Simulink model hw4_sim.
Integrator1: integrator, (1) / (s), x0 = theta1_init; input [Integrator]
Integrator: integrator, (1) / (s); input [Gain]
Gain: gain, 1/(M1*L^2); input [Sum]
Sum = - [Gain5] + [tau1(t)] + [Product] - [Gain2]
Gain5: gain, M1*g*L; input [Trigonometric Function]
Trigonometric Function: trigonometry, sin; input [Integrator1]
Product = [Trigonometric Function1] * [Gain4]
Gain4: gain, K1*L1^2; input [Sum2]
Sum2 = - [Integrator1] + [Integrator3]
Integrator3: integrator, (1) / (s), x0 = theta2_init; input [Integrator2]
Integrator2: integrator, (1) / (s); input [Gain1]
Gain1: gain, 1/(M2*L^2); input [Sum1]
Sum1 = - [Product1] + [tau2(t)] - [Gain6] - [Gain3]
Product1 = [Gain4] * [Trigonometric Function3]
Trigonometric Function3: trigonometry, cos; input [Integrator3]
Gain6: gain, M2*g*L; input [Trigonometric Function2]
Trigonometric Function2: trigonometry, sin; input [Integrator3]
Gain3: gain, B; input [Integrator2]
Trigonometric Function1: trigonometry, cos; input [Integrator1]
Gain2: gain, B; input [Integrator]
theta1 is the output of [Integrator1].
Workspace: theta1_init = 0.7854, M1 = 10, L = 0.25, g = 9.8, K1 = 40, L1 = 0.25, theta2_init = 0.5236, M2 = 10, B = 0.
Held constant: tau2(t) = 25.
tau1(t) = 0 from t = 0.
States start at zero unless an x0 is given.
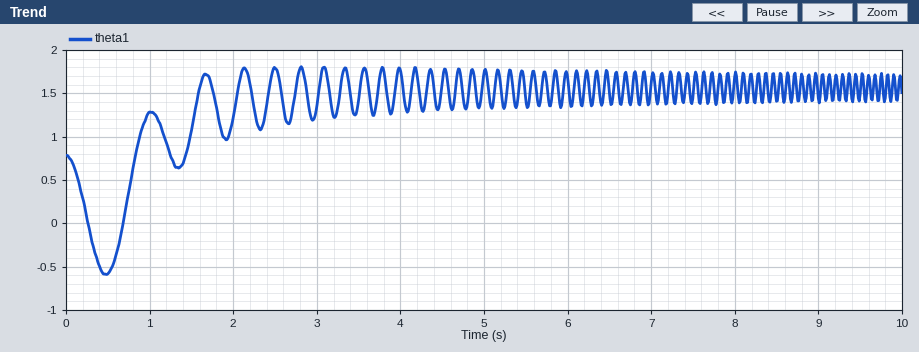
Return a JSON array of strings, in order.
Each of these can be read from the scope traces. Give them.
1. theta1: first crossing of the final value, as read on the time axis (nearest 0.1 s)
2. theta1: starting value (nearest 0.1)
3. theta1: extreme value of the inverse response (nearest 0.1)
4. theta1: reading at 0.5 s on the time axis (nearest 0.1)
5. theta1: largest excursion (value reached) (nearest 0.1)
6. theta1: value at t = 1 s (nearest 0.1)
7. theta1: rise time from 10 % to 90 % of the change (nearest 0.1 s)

["1.6 s", "0.8", "-0.6", "-0.6", "1.8", "1.3", "0.7 s"]
